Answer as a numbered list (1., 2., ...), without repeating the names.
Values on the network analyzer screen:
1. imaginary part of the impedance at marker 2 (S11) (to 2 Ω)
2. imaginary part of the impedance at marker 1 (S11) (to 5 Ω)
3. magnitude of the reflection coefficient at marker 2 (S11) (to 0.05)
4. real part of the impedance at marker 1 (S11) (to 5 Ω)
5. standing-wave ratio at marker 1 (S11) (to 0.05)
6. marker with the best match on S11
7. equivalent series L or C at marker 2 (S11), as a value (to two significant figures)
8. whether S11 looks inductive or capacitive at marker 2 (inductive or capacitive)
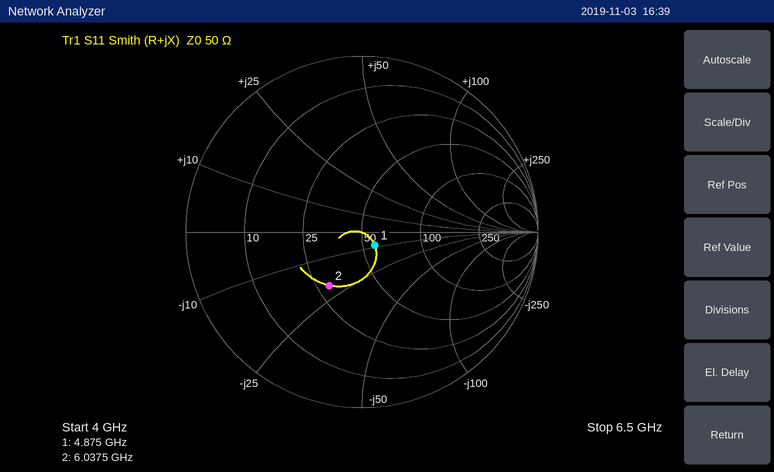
1. -20 Ω
2. -10 Ω
3. 0.35
4. 55 Ω
5. 1.25
6. marker 1
7. 1.3 pF
8. capacitive
